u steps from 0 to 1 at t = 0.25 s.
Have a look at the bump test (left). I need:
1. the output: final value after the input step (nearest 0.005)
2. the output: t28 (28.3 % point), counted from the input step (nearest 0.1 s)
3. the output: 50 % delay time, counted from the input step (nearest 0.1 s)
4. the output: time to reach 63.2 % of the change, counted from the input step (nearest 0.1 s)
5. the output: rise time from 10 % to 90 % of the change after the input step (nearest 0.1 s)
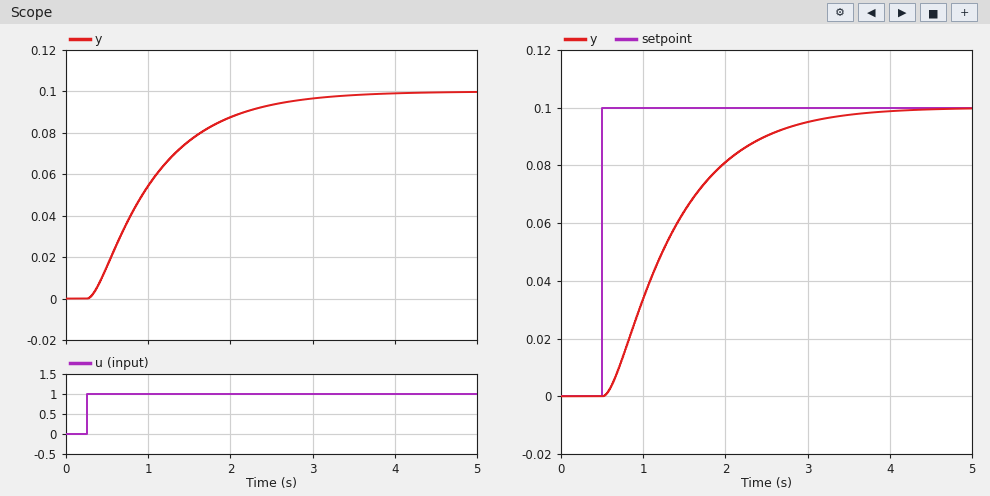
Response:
0.100
0.4 s
0.7 s
0.9 s
1.7 s
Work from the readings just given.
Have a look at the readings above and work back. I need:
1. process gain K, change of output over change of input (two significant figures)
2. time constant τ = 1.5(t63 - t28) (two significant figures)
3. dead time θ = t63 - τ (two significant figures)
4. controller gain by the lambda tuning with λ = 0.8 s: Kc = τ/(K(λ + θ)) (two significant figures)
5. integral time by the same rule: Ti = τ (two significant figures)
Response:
0.10
0.75 s
0.15 s
7.9
0.75 s
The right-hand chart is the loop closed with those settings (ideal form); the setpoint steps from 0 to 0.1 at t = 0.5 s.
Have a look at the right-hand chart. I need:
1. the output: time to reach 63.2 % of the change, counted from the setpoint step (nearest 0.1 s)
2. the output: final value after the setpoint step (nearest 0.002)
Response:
1.0 s
0.100
